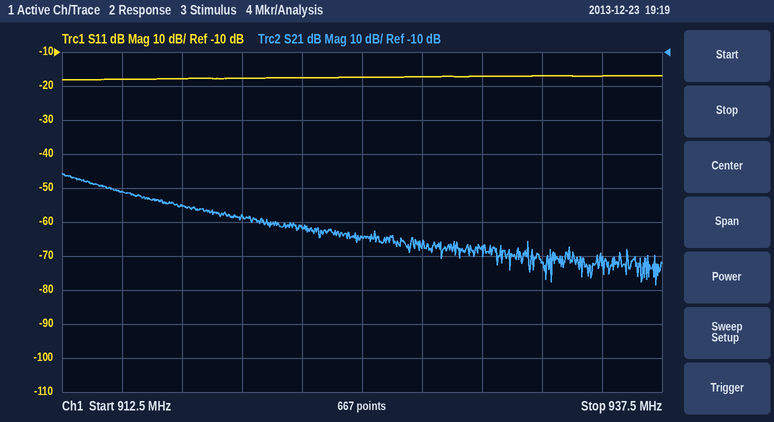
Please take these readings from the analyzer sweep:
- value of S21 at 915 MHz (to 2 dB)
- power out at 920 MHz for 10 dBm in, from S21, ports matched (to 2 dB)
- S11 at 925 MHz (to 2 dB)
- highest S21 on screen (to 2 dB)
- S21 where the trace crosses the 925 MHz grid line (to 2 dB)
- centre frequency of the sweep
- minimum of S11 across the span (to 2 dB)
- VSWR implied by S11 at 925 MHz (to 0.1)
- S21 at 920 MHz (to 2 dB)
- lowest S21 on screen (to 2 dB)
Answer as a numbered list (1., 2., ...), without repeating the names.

1. -52 dB
2. -48 dBm
3. -18 dB
4. -46 dB
5. -64 dB
6. 925 MHz
7. -18 dB
8. 1.3
9. -58 dB
10. -78 dB
